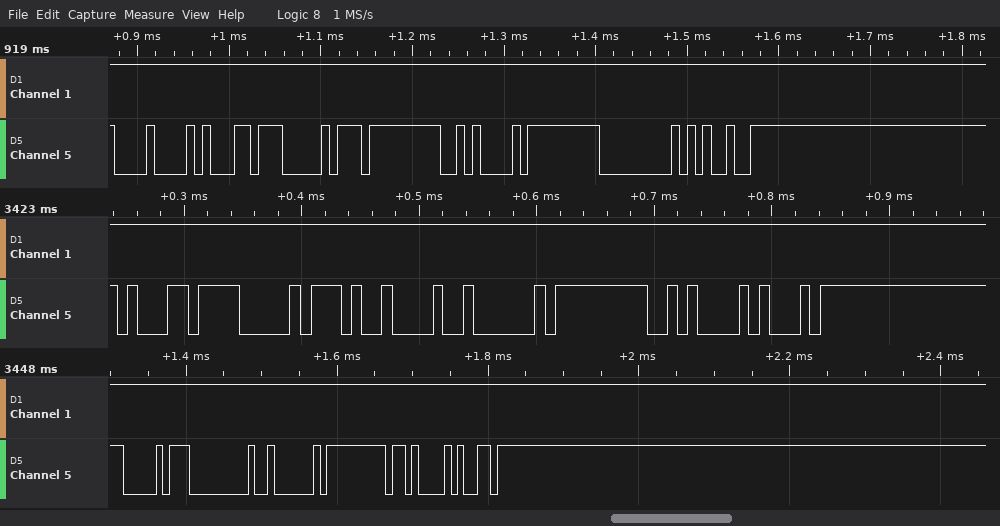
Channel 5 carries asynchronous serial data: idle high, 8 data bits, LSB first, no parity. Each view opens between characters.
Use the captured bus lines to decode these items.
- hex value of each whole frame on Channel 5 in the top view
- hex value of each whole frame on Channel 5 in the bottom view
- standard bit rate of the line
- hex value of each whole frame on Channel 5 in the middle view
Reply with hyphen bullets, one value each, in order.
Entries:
- 08, B1, D0, FF, 0A, FF, 00, 25
- D0, 00, 02, FF, 0B, D9
- 115200 baud
- B1, D0, 09, 02, FF, 0A, D1
